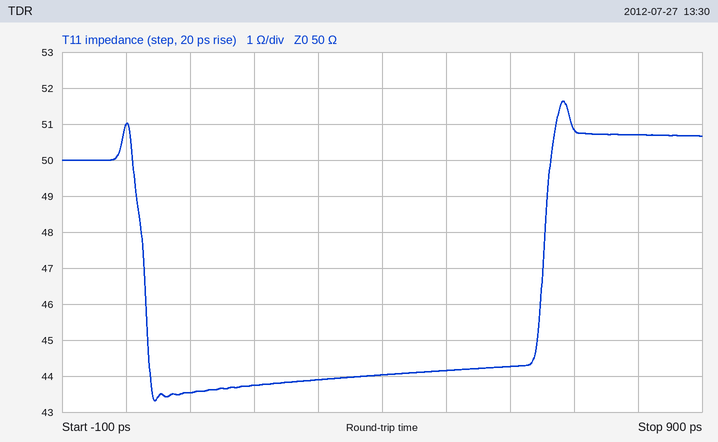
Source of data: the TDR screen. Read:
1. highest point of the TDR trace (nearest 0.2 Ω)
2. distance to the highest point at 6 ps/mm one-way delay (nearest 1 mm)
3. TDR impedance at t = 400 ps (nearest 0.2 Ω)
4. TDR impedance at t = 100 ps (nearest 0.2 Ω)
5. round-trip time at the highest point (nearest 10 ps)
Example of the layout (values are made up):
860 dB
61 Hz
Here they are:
51.6 Ω
57 mm
44.0 Ω
43.6 Ω
680 ps
